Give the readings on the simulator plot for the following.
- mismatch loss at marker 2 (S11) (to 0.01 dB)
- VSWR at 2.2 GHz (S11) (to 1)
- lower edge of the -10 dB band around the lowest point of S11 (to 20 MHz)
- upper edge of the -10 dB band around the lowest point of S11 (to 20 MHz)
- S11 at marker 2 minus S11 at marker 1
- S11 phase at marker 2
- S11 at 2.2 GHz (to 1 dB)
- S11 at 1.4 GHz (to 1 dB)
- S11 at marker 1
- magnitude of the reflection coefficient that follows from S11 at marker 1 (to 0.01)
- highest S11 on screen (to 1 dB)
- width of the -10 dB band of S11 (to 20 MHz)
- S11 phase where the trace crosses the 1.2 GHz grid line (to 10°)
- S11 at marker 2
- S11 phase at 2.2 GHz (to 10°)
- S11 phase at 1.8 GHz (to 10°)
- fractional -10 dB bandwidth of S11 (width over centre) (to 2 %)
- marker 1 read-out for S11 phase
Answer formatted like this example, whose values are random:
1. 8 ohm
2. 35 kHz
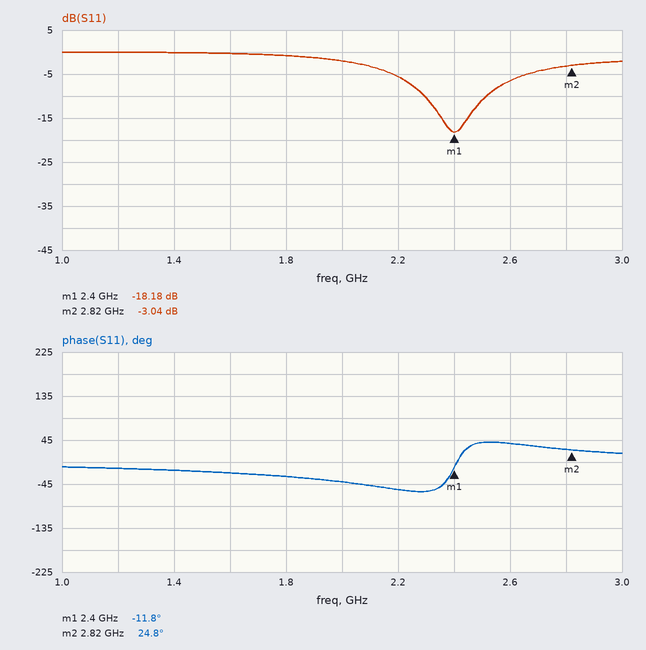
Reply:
1. 2.98 dB
2. 3
3. 2.30 GHz
4. 2.52 GHz
5. 15.14 dB
6. 24.8°
7. -6 dB
8. 0 dB
9. -18.18 dB
10. 0.12
11. 0 dB
12. 220 MHz
13. -10°
14. -3.04 dB
15. -60°
16. -30°
17. 10 %
18. -11.8°
